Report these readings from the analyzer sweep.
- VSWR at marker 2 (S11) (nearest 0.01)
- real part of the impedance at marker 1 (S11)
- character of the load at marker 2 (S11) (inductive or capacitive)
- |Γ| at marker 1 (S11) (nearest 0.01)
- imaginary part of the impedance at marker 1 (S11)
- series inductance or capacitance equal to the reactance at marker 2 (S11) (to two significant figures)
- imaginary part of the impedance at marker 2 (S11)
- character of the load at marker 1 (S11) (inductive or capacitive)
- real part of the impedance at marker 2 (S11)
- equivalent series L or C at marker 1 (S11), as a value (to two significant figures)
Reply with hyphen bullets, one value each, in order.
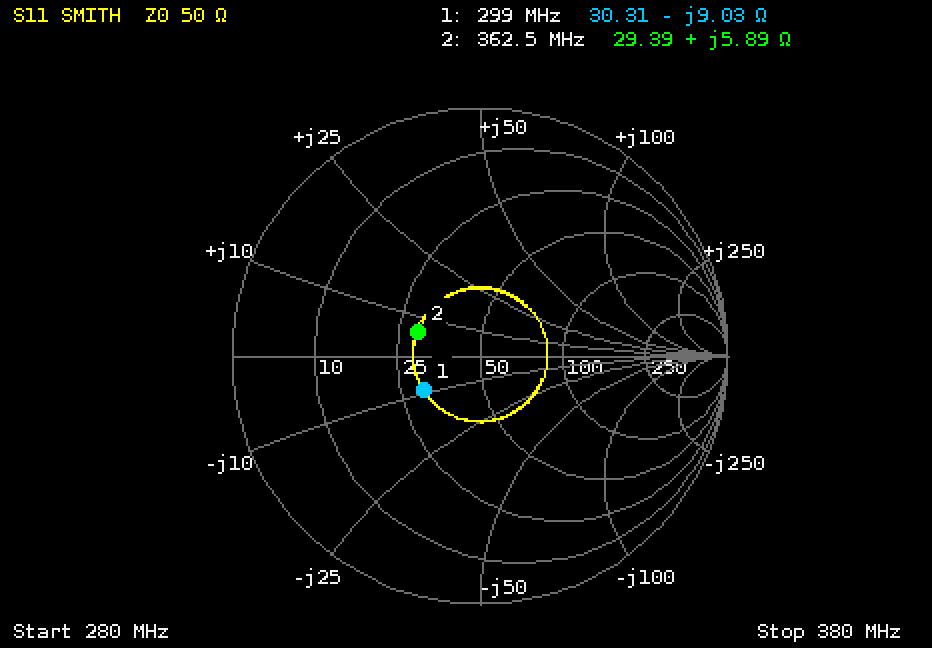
- 1.74
- 30.31 Ω
- inductive
- 0.27
- -9.03 Ω
- 2.6 nH
- +5.89 Ω
- capacitive
- 29.39 Ω
- 59 pF
